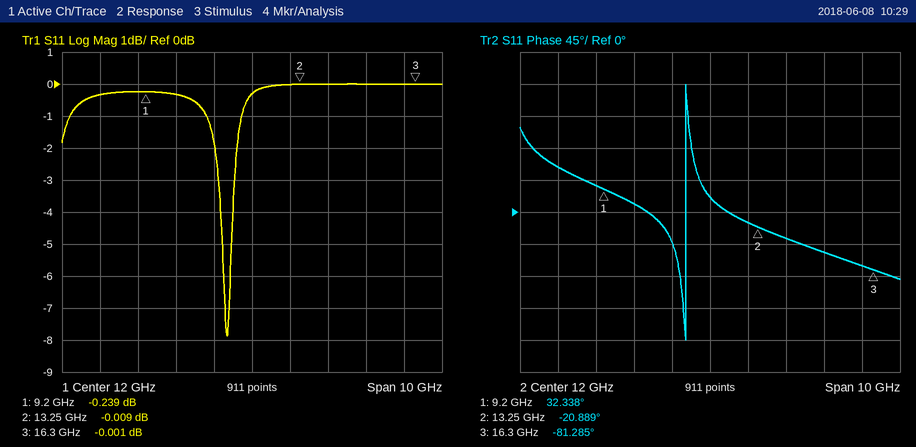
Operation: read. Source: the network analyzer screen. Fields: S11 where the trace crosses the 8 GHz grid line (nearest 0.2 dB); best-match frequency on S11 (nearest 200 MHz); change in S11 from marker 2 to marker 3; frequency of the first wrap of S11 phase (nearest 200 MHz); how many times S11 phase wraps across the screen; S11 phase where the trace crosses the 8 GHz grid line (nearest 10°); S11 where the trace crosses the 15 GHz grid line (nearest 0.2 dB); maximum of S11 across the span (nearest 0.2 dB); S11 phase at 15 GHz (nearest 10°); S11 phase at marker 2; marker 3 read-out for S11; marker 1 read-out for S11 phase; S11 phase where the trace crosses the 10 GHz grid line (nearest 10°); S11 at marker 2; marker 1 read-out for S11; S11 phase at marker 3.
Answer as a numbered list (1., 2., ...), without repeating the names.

1. -0.4 dB
2. 11.4 GHz
3. 0.008 dB
4. 11.4 GHz
5. 1
6. 60°
7. 0.0 dB
8. 0.0 dB
9. -60°
10. -20.889°
11. -0.001 dB
12. 32.338°
13. 10°
14. -0.009 dB
15. -0.239 dB
16. -81.285°
